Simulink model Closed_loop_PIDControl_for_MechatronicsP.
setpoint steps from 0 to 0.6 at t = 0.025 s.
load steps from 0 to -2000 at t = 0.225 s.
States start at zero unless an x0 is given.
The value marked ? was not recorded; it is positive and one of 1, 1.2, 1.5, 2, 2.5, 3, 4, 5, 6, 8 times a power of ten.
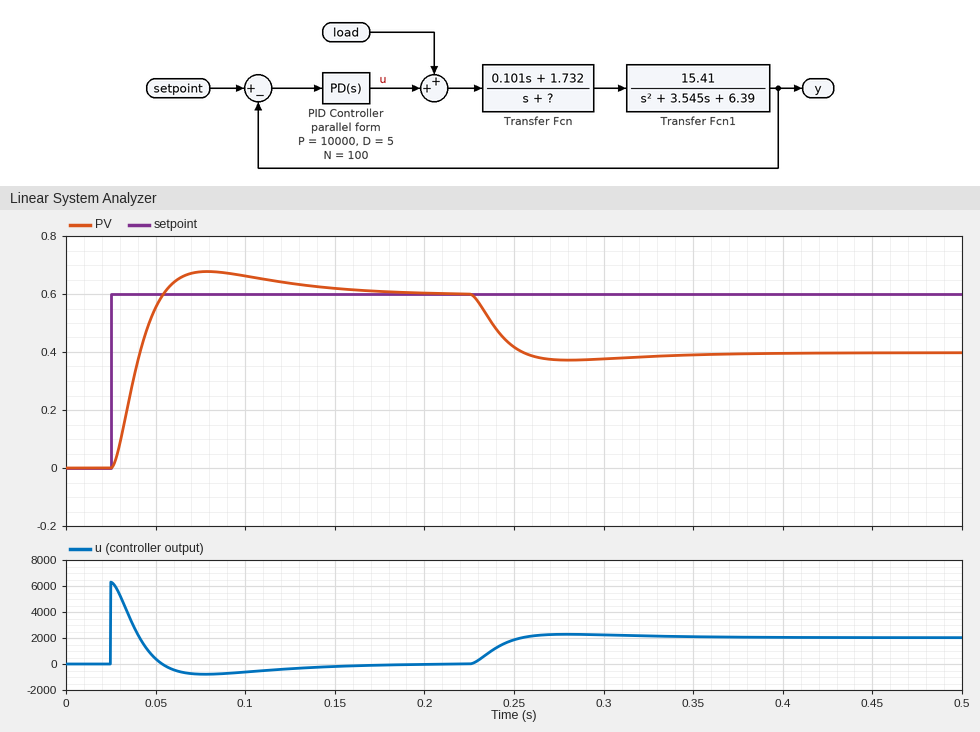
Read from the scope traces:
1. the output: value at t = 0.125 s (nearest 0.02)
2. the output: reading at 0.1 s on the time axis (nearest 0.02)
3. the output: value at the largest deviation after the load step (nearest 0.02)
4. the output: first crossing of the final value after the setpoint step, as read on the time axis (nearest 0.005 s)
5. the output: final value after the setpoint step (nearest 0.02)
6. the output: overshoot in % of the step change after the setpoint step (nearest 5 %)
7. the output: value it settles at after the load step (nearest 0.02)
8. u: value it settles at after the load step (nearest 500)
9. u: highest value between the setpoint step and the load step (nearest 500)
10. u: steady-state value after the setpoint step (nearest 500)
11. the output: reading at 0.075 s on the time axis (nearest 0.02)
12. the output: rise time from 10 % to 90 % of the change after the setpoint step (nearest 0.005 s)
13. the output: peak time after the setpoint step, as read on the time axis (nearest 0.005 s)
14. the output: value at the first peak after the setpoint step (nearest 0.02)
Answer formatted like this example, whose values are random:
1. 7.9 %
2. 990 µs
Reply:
1. 0.64
2. 0.66
3. 0.38
4. 0.055 s
5. 0.60
6. 15 %
7. 0.40
8. 2000
9. 6500
10. 0
11. 0.68
12. 0.020 s
13. 0.080 s
14. 0.68
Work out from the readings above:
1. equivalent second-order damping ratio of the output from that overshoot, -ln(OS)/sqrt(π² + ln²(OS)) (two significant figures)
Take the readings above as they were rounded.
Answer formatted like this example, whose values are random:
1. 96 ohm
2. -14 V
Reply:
1. 0.52
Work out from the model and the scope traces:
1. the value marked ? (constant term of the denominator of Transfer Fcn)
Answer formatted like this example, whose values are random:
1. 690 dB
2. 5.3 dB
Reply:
1. 250
